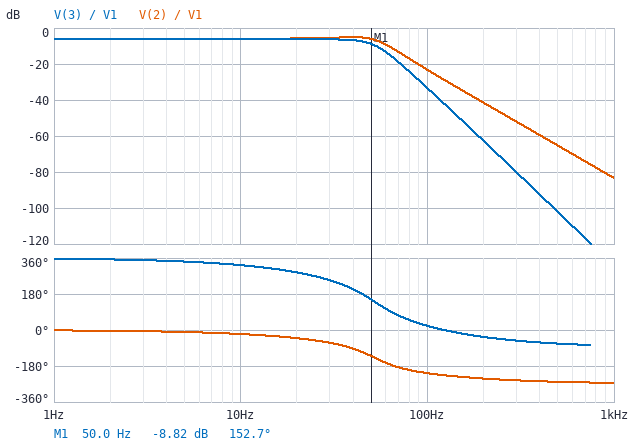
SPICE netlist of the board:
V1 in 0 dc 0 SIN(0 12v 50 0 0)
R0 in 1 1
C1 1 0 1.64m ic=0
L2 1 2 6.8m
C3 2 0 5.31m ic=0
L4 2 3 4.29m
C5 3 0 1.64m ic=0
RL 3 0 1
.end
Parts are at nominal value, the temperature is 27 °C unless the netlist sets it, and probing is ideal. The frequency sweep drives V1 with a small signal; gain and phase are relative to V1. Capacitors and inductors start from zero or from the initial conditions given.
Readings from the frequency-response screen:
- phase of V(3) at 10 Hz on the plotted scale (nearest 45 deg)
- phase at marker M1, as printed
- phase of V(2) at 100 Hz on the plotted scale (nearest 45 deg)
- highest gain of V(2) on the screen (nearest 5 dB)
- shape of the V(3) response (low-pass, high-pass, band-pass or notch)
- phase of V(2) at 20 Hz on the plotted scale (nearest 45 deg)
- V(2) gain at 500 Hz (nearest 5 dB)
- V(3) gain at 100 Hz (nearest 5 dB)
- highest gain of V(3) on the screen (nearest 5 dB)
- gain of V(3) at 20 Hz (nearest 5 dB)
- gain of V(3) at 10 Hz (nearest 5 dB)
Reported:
315 deg
152.7 deg
-225 deg
-5 dB
low-pass
-45 deg
-65 dB
-35 dB
-5 dB
-5 dB
-5 dB
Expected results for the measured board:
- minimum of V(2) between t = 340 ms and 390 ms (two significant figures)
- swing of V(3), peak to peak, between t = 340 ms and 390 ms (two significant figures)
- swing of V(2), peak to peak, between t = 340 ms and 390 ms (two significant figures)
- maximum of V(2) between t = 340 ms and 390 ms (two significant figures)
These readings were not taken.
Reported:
-6.0 V
8.7 V
12 V
6.0 V
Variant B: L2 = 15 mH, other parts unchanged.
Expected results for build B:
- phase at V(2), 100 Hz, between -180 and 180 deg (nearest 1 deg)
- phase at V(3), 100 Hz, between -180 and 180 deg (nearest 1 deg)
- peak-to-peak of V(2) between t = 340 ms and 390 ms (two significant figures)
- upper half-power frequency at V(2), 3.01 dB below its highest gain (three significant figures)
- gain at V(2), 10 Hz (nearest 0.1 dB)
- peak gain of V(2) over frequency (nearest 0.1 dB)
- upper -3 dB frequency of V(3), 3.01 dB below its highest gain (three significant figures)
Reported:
139 deg
16 deg
4.9 V
32.1 Hz
-6.4 dB
-6.0 dB
27.4 Hz
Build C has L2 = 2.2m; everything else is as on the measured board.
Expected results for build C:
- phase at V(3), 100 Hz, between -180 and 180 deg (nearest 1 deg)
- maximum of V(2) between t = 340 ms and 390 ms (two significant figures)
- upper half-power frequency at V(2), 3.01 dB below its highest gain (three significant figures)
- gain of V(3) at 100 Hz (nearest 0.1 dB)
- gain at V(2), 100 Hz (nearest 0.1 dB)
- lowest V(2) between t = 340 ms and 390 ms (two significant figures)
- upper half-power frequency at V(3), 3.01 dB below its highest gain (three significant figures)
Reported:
55 deg
7.2 V
90.0 Hz
-19.9 dB
-9.7 dB
-7.2 V
65.0 Hz
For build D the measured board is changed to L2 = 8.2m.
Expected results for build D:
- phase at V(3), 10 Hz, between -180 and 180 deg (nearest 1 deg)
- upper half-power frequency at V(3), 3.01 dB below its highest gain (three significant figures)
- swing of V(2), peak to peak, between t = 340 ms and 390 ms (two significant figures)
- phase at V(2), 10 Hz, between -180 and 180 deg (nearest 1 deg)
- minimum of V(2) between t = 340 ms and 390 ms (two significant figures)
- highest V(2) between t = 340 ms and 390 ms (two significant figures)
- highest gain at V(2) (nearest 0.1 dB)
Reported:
-38 deg
46.1 Hz
10 V
-23 deg
-5.0 V
5.0 V
-5.8 dB
